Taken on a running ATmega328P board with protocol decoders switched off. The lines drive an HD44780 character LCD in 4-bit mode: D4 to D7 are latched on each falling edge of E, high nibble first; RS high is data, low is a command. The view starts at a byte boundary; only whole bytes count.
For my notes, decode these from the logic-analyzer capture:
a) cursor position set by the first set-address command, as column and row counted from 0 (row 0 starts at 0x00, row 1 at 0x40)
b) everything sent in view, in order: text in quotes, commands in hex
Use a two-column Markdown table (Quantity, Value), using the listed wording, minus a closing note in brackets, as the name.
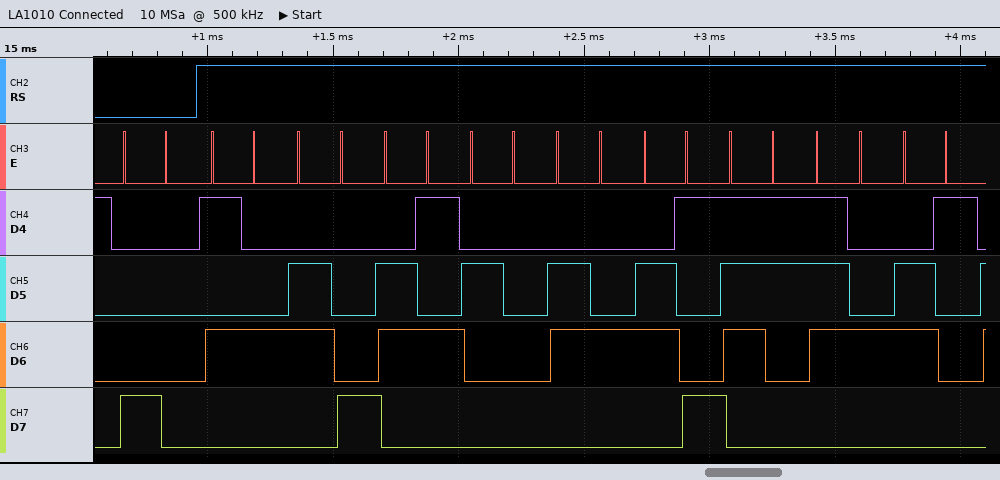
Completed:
| Quantity | Value |
|---|---|
| cursor position set by the first set-address command, as column and row counted from 0 | column 0, row 0 |
| everything sent in view, in order: text in quotes, commands in hex | 0x80 "The dista" |
